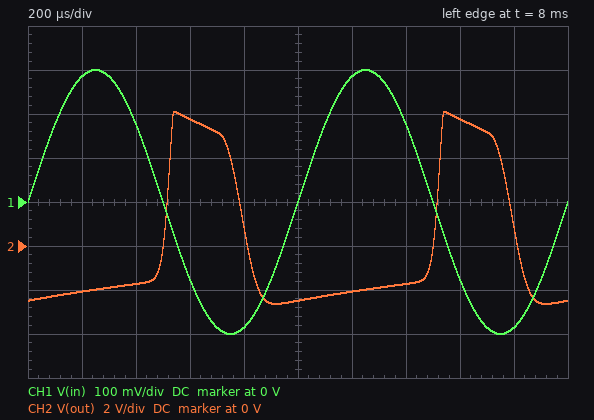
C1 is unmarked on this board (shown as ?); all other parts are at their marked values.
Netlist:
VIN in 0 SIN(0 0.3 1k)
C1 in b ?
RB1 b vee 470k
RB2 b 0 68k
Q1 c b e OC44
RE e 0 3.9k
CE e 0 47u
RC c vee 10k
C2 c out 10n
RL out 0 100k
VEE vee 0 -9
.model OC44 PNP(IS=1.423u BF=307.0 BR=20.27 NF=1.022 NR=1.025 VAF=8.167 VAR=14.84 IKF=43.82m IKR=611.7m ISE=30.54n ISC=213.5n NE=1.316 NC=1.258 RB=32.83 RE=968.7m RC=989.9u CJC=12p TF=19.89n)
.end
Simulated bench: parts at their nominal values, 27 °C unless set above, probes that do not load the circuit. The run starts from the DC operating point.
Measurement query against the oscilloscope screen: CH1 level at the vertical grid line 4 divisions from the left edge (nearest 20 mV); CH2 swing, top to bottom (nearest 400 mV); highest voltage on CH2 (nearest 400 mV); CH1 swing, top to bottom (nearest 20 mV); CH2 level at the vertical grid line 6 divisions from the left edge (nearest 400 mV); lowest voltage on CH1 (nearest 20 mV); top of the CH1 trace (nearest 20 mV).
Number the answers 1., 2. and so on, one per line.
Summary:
1. -280 mV
2. 8.8 V
3. 6.0 V
4. 600 mV
5. -2.0 V
6. -300 mV
7. 300 mV
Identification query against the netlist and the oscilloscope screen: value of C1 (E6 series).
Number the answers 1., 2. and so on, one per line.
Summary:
1. 15 nF
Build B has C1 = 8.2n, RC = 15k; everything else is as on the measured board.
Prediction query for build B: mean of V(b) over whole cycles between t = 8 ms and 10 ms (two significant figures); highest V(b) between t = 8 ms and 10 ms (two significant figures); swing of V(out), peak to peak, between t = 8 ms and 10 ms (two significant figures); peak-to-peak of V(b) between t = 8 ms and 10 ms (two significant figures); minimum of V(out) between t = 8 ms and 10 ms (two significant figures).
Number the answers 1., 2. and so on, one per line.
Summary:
1. -940 mV
2. -720 mV
3. 8.6 V
4. 370 mV
5. -3.1 V
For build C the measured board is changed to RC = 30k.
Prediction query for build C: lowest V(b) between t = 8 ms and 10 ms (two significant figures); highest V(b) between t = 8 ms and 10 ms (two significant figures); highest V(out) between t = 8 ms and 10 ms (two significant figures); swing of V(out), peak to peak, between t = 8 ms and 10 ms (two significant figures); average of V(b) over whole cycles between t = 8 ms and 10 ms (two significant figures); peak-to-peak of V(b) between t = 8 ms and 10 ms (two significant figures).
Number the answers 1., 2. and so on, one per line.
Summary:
1. -1.0 V
2. -600 mV
3. 5.5 V
4. 8.3 V
5. -850 mV
6. 440 mV
